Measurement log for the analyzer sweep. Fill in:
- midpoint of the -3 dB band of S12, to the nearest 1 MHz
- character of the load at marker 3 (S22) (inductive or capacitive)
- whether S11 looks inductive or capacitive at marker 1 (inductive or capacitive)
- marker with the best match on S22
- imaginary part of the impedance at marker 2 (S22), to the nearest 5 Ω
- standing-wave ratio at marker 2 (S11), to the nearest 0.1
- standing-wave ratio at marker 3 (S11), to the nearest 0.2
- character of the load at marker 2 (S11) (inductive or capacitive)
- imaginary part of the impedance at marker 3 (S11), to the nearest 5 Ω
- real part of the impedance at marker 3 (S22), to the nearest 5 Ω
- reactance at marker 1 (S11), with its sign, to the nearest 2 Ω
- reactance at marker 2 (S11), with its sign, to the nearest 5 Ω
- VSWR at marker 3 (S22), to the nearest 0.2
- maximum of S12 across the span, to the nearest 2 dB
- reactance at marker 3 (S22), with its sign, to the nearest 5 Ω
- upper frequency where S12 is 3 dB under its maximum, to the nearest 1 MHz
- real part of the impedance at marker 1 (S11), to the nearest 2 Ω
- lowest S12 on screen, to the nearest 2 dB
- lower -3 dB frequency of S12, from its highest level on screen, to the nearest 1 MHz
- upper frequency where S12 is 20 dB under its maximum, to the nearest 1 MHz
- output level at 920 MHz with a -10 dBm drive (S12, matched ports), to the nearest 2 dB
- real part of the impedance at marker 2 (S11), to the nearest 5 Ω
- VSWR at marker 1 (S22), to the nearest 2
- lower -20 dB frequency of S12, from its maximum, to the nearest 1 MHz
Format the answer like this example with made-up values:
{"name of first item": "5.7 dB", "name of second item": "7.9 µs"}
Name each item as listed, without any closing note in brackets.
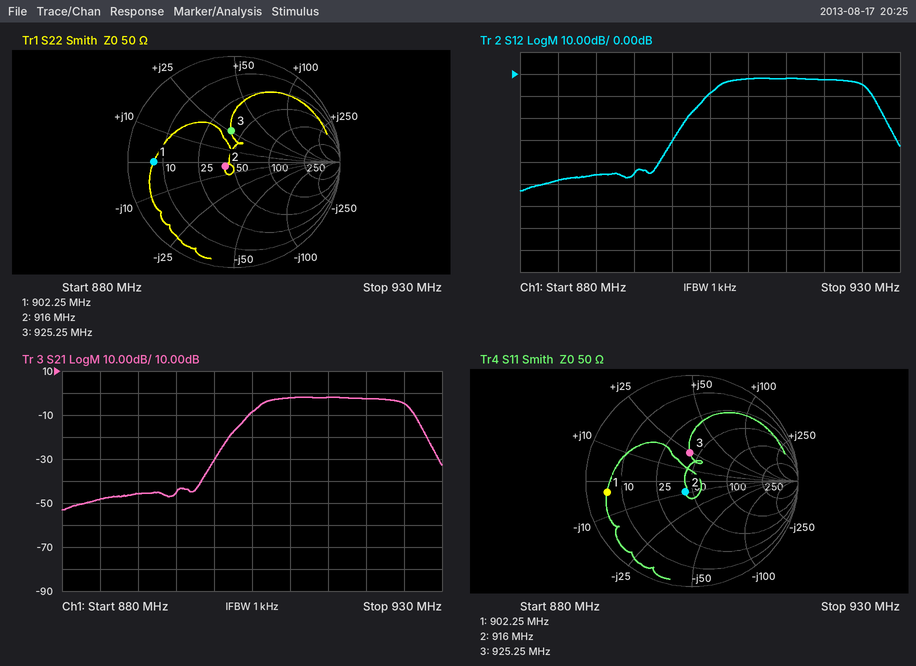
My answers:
{"midpoint of the -3 dB band of S12, to the nearest 1 MHz": "916 MHz", "character of the load at marker 3 (S22)": "inductive", "whether S11 looks inductive or capacitive at marker 1": "capacitive", "marker with the best match on S22": "marker 2", "imaginary part of the impedance at marker 2 (S22), to the nearest 5 Ω": "-5 Ω", "standing-wave ratio at marker 2 (S11), to the nearest 0.1": "1.3", "standing-wave ratio at marker 3 (S11), to the nearest 0.2": "1.8", "character of the load at marker 2 (S11)": "capacitive", "imaginary part of the impedance at marker 3 (S11), to the nearest 5 Ω": "+25 Ω", "real part of the impedance at marker 3 (S22), to the nearest 5 Ω": "40 Ω", "reactance at marker 1 (S11), with its sign, to the nearest 2 Ω": "-4 Ω", "reactance at marker 2 (S11), with its sign, to the nearest 5 Ω": "-10 Ω", "VSWR at marker 3 (S22), to the nearest 0.2": "1.8", "maximum of S12 across the span, to the nearest 2 dB": "-2 dB", "reactance at marker 3 (S22), with its sign, to the nearest 5 Ω": "+25 Ω", "upper frequency where S12 is 3 dB under its maximum, to the nearest 1 MHz": "925 MHz", "real part of the impedance at marker 1 (S11), to the nearest 2 Ω": "6 Ω", "lowest S12 on screen, to the nearest 2 dB": "-54 dB", "lower -3 dB frequency of S12, from its highest level on screen, to the nearest 1 MHz": "906 MHz", "upper frequency where S12 is 20 dB under its maximum, to the nearest 1 MHz": "928 MHz", "output level at 920 MHz with a -10 dBm drive (S12, matched ports), to the nearest 2 dB": "-12 dBm", "real part of the impedance at marker 2 (S11), to the nearest 5 Ω": "45 Ω", "VSWR at marker 1 (S22), to the nearest 2": "8", "lower -20 dB frequency of S12, from its maximum, to the nearest 1 MHz": "902 MHz"}
